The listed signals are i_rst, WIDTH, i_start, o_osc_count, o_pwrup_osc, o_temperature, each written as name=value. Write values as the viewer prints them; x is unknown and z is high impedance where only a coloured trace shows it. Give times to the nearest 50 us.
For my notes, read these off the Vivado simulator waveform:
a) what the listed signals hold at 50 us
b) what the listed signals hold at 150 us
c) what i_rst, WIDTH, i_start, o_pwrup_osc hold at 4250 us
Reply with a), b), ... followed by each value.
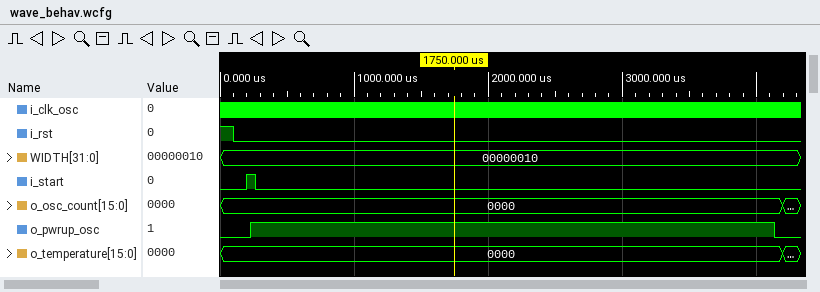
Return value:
a) i_rst=1, WIDTH=00000010, i_start=0, o_osc_count=0000, o_pwrup_osc=0, o_temperature=0000
b) i_rst=0, WIDTH=00000010, i_start=0, o_osc_count=0000, o_pwrup_osc=0, o_temperature=0000
c) i_rst=0, WIDTH=00000010, i_start=0, o_pwrup_osc=0
